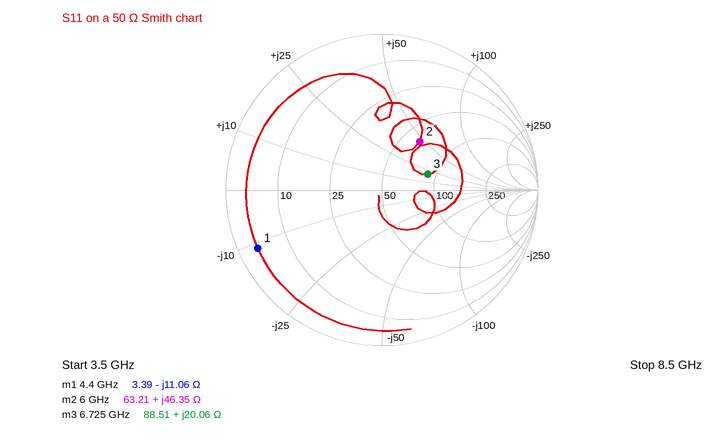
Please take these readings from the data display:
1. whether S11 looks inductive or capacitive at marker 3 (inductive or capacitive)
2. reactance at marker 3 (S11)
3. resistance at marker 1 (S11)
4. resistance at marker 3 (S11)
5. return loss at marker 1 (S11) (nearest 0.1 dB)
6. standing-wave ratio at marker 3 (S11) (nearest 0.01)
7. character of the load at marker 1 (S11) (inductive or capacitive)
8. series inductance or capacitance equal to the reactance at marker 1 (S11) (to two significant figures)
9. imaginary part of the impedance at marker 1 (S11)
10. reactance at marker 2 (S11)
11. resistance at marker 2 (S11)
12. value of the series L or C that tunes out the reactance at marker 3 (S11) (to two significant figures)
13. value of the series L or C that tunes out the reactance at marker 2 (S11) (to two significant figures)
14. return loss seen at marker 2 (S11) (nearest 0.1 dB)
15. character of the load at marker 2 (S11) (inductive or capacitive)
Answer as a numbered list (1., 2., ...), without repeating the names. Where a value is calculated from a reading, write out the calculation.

1. inductive
2. +20.06 Ω
3. 3.39 Ω
4. 88.51 Ω
5. 1.1 dB
6. 1.90
7. capacitive
8. C = 1/(2π × 4.4 GHz × 11.06 Ω) ≈ 3.3 pF
9. -11.06 Ω
10. +46.35 Ω
11. 63.21 Ω
12. C = 1/(2π × 6.725 GHz × 20.06 Ω) ≈ 1.2 pF
13. C = 1/(2π × 6 GHz × 46.35 Ω) ≈ 572 fF, so 570 fF to two significant figures
14. 8.1 dB
15. inductive
